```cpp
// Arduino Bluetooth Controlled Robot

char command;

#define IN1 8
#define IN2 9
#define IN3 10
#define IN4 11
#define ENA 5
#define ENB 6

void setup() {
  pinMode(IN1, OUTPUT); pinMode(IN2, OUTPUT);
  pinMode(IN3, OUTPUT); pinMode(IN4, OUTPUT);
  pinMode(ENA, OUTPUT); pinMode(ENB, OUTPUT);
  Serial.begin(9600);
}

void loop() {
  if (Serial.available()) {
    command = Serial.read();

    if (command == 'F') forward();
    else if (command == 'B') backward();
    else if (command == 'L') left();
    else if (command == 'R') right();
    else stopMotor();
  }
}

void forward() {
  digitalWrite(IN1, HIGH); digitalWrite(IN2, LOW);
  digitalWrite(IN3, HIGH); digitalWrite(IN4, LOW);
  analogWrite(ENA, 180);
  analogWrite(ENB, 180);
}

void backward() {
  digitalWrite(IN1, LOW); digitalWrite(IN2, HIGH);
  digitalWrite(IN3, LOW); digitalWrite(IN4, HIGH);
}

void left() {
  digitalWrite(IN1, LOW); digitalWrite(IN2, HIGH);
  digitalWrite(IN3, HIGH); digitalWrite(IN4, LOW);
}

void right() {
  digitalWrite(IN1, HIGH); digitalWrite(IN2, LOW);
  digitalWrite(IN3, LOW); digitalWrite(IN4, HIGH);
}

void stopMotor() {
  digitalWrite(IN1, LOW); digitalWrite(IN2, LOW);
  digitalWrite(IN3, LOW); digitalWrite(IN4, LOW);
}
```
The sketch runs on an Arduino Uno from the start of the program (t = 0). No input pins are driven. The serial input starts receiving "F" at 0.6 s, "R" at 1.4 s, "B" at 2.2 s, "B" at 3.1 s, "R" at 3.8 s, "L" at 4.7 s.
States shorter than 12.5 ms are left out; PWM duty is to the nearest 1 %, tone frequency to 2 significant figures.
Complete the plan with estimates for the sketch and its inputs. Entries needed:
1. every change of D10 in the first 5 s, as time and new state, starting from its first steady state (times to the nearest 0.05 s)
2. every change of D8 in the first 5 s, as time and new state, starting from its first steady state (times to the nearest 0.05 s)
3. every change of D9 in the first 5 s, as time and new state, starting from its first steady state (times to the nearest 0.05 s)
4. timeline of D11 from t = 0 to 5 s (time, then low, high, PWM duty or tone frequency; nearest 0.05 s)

0 s low; 0.6 s high; 1.4 s low; 4.7 s high
0 s low; 0.6 s high; 2.2 s low; 3.8 s high; 4.7 s low
0 s low; 2.2 s high; 3.8 s low; 4.7 s high
0 s low; 1.4 s high; 4.7 s low
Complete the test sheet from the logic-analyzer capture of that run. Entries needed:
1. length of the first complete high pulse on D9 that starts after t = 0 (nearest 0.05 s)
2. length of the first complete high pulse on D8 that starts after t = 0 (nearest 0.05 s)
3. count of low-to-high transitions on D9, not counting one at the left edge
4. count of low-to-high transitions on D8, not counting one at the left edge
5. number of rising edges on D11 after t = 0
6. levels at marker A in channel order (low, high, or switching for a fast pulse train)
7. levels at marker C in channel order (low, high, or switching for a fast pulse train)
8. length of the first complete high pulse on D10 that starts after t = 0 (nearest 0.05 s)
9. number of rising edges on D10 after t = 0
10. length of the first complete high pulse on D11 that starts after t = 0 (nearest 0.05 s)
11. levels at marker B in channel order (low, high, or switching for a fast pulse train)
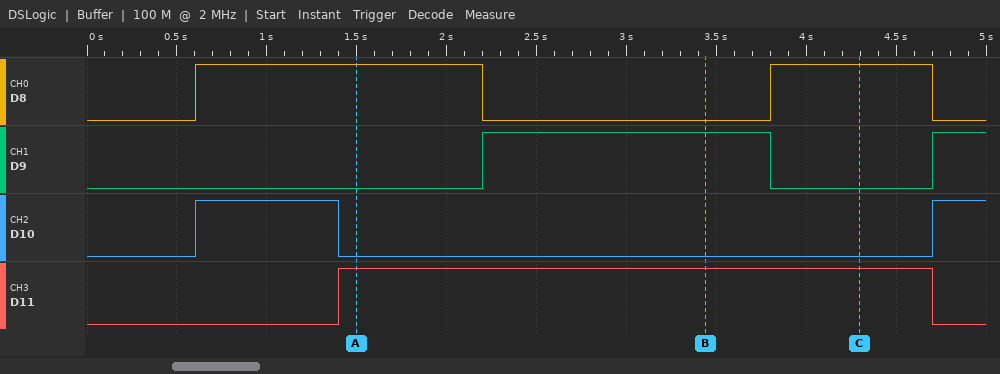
1.60 s
1.60 s
2
2
1
D8 high, D9 low, D10 low, D11 high
D8 high, D9 low, D10 low, D11 high
0.80 s
2
3.30 s
D8 low, D9 high, D10 low, D11 high
